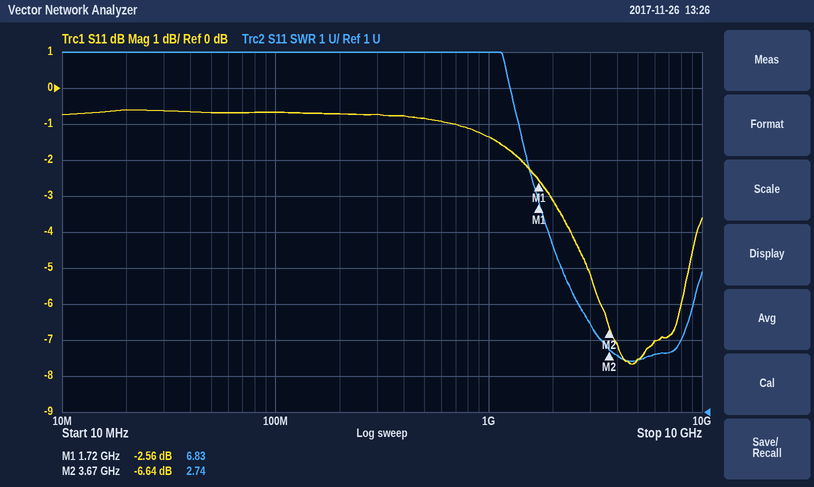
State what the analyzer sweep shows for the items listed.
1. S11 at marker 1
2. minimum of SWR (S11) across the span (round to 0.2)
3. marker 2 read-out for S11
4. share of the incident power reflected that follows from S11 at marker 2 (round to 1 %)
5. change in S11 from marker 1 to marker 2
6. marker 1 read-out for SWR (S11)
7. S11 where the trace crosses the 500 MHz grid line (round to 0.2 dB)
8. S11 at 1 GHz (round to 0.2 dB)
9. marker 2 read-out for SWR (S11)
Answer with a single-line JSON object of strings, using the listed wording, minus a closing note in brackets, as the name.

{"S11 at marker 1": "-2.56 dB", "minimum of SWR (S11) across the span": "2.4", "marker 2 read-out for S11": "-6.64 dB", "share of the incident power reflected that follows from S11 at marker 2": "22 %", "change in S11 from marker 1 to marker 2": "-4.08 dB", "marker 1 read-out for SWR": "6.83", "S11 where the trace crosses the 500 MHz grid line": "-0.8 dB", "S11 at 1 GHz": "-1.4 dB", "marker 2 read-out for SWR": "2.74"}
